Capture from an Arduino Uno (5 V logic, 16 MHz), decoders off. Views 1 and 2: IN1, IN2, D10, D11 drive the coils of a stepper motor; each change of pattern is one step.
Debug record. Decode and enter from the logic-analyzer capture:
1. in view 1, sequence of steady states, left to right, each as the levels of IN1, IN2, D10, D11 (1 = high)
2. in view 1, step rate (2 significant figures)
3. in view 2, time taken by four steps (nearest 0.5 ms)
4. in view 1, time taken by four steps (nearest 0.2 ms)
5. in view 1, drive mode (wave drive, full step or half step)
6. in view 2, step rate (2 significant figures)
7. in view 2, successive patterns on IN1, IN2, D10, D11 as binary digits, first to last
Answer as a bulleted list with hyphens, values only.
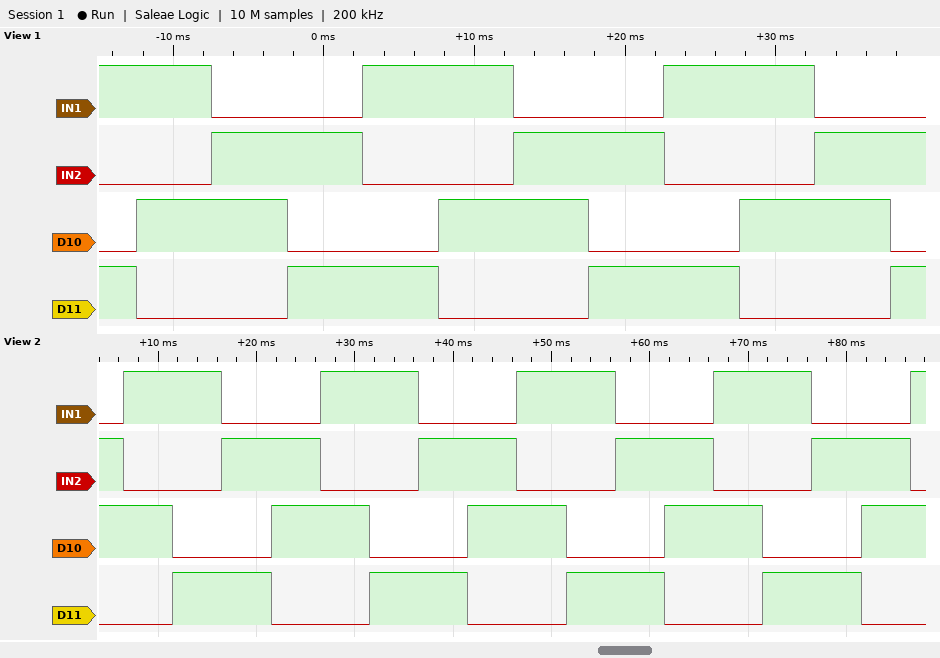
- 1001 1010 0110 0101 1001 1010 0110 0101 1001 1010 0110 0101
- 200 steps/s
- 20.0 ms
- 20.0 ms
- full step
- 200 steps/s
- 0110 1010 1001 0101 0110 1010 1001 0101 0110 1010 1001 0101 0110 1010 1001 0101 0110 1010
